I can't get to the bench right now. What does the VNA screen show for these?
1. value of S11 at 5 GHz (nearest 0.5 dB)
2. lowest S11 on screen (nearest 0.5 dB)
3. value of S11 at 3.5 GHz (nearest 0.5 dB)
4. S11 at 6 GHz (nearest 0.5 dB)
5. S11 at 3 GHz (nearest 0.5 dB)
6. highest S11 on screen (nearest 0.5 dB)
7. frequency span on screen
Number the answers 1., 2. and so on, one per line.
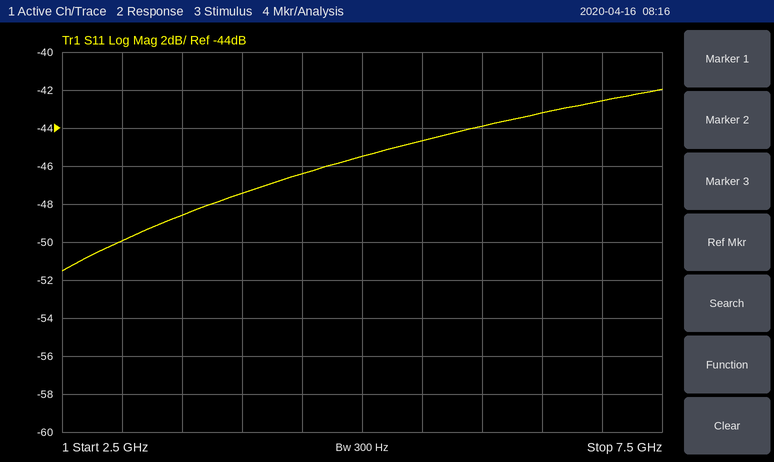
1. -45.5 dB
2. -51.5 dB
3. -48.5 dB
4. -44.0 dB
5. -50.0 dB
6. -42.0 dB
7. 5 GHz
